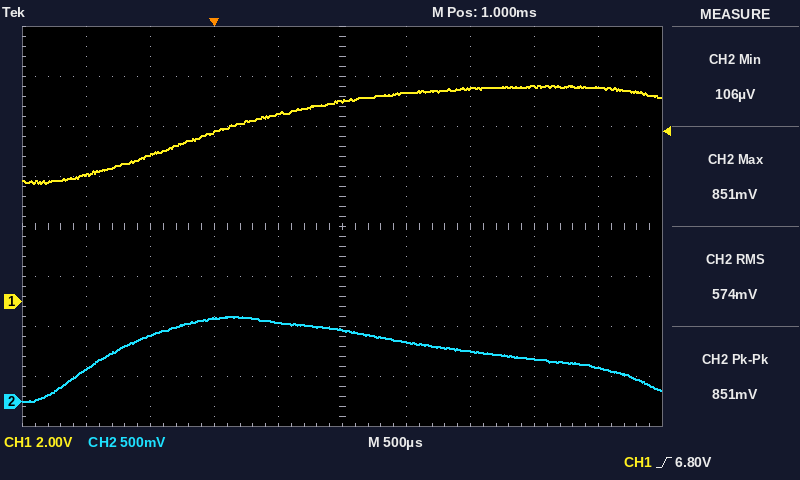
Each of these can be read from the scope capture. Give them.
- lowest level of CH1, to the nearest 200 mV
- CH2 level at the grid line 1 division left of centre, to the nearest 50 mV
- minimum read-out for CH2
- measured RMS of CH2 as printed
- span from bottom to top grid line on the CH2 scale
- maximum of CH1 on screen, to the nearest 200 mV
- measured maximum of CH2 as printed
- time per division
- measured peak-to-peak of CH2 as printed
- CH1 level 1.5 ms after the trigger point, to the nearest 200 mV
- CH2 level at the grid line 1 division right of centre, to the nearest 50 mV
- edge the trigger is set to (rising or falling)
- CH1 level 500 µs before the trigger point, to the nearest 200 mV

4.8 V
800 mV
106 µV
574 mV
4 V
8.6 V
851 mV
500 µs
851 mV
8.4 V
600 mV
rising
5.8 V
